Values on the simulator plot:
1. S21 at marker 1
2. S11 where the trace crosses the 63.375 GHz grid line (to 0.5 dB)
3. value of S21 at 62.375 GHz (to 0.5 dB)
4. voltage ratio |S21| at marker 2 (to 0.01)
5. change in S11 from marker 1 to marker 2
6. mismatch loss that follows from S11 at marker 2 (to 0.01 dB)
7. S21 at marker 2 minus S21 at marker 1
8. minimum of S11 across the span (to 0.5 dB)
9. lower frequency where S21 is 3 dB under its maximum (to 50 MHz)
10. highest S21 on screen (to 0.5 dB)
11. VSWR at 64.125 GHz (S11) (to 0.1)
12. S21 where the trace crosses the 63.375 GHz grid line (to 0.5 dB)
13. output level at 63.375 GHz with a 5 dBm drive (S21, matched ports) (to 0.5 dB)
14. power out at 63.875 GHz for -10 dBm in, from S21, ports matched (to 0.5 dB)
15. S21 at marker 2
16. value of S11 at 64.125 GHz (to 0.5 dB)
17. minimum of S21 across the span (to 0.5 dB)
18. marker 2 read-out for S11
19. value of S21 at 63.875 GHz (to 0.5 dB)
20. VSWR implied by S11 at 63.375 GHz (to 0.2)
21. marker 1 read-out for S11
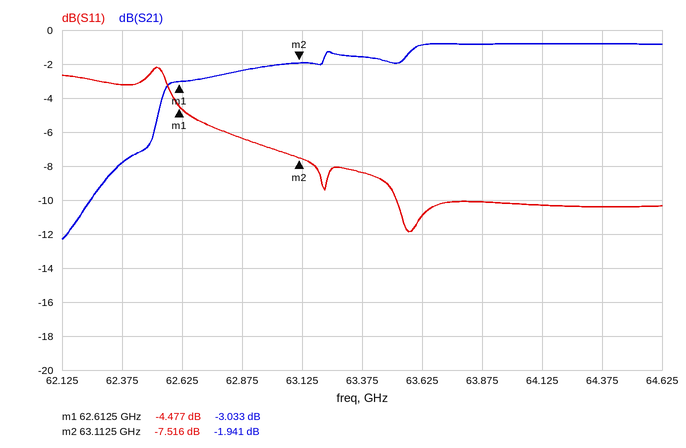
-3.033 dB
-8.5 dB
-8.0 dB
0.80
-3.039 dB
0.85 dB
1.092 dB
-12.0 dB
62.55 GHz
-1.0 dB
1.9
-1.5 dB
3.5 dBm
-11.0 dBm
-1.941 dB
-10.5 dB
-12.5 dB
-7.516 dB
-1.0 dB
2.2
-4.477 dB
